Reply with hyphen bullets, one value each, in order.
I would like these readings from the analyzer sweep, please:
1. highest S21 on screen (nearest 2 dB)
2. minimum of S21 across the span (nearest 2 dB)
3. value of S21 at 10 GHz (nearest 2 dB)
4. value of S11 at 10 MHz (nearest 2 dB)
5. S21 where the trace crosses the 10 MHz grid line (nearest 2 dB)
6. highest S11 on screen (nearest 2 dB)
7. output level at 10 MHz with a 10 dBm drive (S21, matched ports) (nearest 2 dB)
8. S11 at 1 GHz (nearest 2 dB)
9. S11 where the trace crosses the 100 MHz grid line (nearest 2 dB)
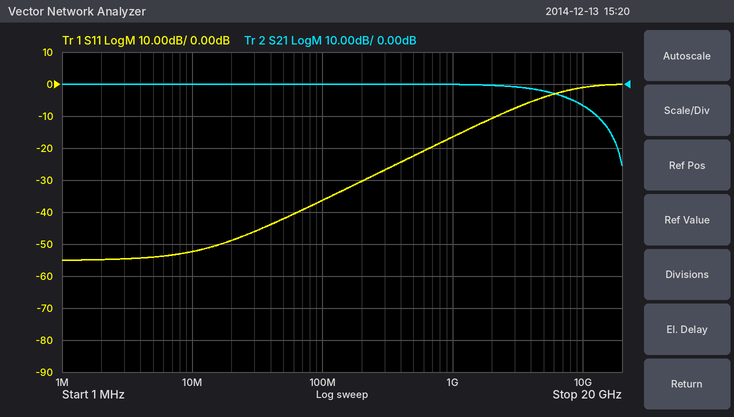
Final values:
- 0 dB
- -26 dB
- -6 dB
- -52 dB
- 0 dB
- 0 dB
- 10 dBm
- -16 dB
- -36 dB
